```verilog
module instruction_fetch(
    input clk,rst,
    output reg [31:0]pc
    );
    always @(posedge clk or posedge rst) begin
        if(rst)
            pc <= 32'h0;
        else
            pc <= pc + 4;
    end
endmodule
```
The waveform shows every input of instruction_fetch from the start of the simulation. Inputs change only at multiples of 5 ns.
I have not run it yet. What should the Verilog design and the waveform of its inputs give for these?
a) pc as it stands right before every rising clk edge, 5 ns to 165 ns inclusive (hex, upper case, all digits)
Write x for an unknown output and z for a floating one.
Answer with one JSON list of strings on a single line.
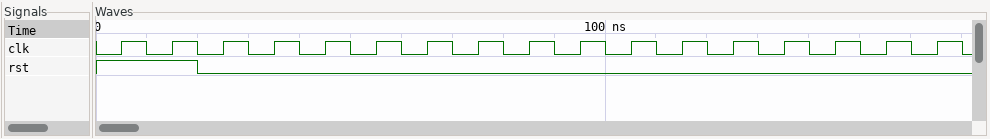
["00000000, 00000000, 00000000, 00000004, 00000008, 0000000C, 00000010, 00000014, 00000018, 0000001C, 00000020, 00000024, 00000028, 0000002C, 00000030, 00000034, 00000038"]
